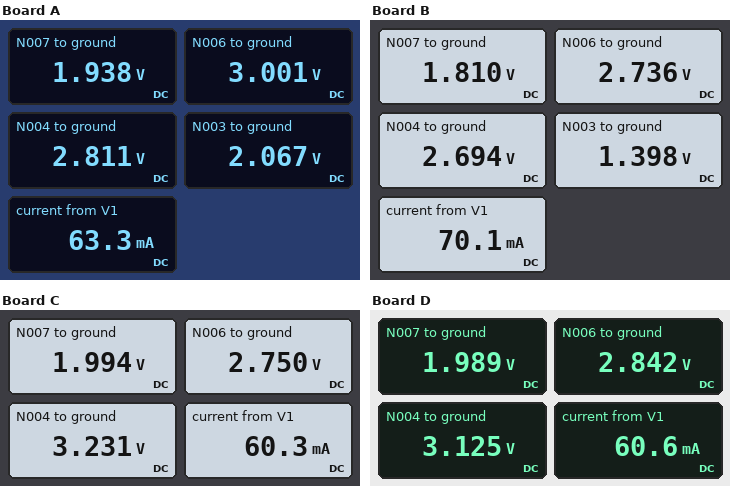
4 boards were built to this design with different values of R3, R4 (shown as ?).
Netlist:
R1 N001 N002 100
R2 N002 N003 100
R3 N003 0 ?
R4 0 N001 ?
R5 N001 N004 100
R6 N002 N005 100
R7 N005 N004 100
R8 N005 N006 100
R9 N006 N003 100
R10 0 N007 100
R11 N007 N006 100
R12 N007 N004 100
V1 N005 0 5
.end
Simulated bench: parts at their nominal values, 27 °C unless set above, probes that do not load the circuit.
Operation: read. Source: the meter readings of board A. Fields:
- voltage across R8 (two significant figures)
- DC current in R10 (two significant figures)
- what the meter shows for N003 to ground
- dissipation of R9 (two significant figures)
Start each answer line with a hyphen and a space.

- 2.0 V
- 19 mA
- 2.067 V
- 8.7 mW
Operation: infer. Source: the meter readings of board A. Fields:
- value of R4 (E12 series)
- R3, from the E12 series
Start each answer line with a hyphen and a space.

- 56 Ω
- 120 Ω
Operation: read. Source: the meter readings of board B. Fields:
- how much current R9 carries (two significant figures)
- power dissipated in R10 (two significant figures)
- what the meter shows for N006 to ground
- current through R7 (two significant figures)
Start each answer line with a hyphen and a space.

- 13 mA
- 33 mW
- 2.736 V
- 23 mA
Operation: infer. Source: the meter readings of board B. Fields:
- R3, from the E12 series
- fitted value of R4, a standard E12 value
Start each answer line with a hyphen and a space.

- 56 Ω
- 47 Ω
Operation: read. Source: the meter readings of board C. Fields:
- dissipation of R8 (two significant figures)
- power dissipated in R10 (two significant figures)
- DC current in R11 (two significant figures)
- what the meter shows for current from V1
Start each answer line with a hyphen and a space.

- 51 mW
- 40 mW
- 7.6 mA
- 60.3 mA
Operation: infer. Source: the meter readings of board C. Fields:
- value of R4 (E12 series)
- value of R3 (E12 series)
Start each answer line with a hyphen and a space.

- 330 Ω
- 39 Ω
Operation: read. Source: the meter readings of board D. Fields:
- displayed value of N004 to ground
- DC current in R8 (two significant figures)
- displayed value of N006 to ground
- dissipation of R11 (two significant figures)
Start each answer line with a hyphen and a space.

- 3.125 V
- 22 mA
- 2.842 V
- 7.3 mW
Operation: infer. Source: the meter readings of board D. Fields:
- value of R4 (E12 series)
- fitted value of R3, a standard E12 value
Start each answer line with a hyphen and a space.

- 180 Ω
- 56 Ω
